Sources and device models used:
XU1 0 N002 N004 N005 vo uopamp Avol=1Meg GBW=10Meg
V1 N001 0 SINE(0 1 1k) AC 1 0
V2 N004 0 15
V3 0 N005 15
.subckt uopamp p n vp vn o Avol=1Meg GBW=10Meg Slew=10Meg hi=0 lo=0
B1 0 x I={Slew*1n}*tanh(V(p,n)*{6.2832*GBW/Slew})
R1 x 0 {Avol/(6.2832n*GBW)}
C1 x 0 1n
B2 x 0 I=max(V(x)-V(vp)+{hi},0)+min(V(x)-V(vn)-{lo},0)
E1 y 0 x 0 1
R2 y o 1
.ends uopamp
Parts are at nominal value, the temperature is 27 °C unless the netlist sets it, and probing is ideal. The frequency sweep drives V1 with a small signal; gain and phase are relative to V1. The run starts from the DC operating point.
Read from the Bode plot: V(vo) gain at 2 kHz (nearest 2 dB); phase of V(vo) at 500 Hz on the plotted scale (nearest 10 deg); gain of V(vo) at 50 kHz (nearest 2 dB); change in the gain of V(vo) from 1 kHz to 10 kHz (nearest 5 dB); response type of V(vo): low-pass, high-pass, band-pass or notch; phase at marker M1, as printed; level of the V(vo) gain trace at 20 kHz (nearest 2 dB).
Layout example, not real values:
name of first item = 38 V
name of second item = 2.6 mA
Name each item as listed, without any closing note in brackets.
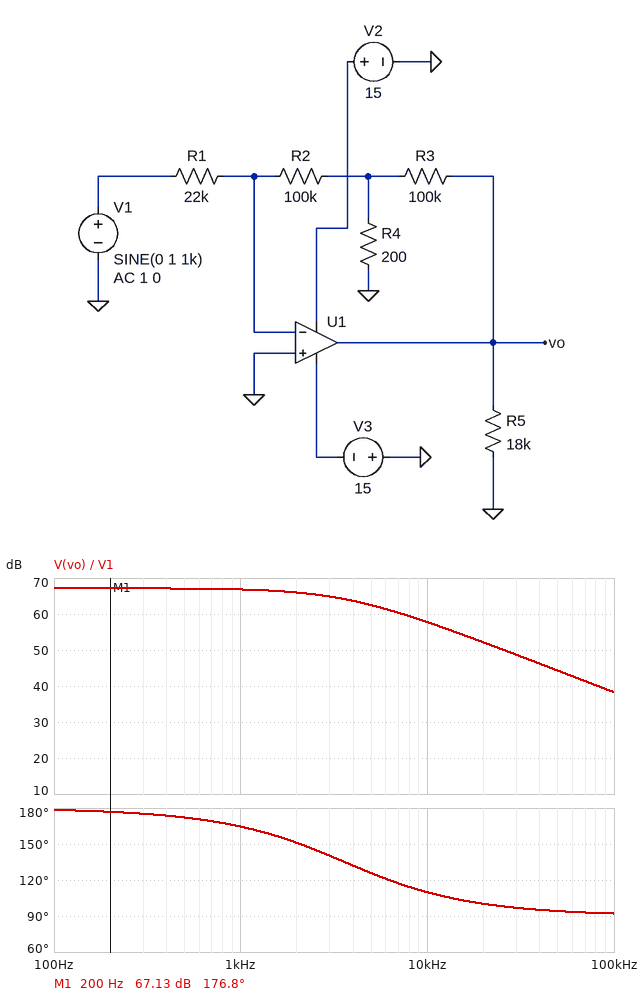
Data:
V(vo) gain at 2 kHz = 66 dB
phase of V(vo) at 500 Hz on the plotted scale = 170 deg
gain of V(vo) at 50 kHz = 44 dB
change in the gain of V(vo) from 1 kHz to 10 kHz = -10 dB
response type of V(vo): low-pass, high-pass, band-pass or notch = low-pass
phase at marker M1, as printed = 176.8 deg
level of the V(vo) gain trace at 20 kHz = 52 dB
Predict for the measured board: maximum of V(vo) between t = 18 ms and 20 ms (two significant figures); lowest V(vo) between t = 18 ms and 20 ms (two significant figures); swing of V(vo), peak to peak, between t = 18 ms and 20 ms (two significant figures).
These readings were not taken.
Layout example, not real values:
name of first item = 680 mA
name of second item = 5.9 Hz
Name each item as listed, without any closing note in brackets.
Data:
maximum of V(vo) between t = 18 ms and 20 ms = 15 V
lowest V(vo) between t = 18 ms and 20 ms = -15 V
swing of V(vo), peak to peak, between t = 18 ms and 20 ms = 30 V
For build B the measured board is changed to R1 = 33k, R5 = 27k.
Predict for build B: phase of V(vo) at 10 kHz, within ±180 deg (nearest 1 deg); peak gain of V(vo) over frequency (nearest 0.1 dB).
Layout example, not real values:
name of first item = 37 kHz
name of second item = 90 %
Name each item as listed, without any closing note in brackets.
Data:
phase of V(vo) at 10 kHz, within ±180 deg = 116 deg
peak gain of V(vo) over frequency = 63.6 dB
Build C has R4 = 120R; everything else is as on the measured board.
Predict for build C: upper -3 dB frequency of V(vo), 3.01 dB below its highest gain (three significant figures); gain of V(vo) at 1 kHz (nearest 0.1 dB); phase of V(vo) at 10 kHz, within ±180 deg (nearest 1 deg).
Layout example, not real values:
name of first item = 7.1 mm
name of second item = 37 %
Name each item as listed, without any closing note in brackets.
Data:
upper -3 dB frequency of V(vo), 3.01 dB below its highest gain = 2.17 kHz
gain of V(vo) at 1 kHz = 70.7 dB
phase of V(vo) at 10 kHz, within ±180 deg = 102 deg
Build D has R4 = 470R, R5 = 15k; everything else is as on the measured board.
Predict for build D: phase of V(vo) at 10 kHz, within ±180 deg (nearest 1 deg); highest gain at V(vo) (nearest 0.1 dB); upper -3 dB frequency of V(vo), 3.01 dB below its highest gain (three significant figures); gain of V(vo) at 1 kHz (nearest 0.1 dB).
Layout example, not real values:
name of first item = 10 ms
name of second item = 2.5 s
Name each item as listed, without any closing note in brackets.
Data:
phase of V(vo) at 10 kHz, within ±180 deg = 130 deg
highest gain at V(vo) = 59.8 dB
upper -3 dB frequency of V(vo), 3.01 dB below its highest gain = 8.41 kHz
gain of V(vo) at 1 kHz = 59.7 dB
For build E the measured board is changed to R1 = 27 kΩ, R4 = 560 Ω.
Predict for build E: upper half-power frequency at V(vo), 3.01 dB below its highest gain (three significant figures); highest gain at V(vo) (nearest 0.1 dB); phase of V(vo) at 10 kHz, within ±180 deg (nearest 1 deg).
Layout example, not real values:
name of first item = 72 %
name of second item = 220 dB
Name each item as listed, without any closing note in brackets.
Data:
upper half-power frequency at V(vo), 3.01 dB below its highest gain = 11.8 kHz
highest gain at V(vo) = 56.5 dB
phase of V(vo) at 10 kHz, within ±180 deg = 140 deg
